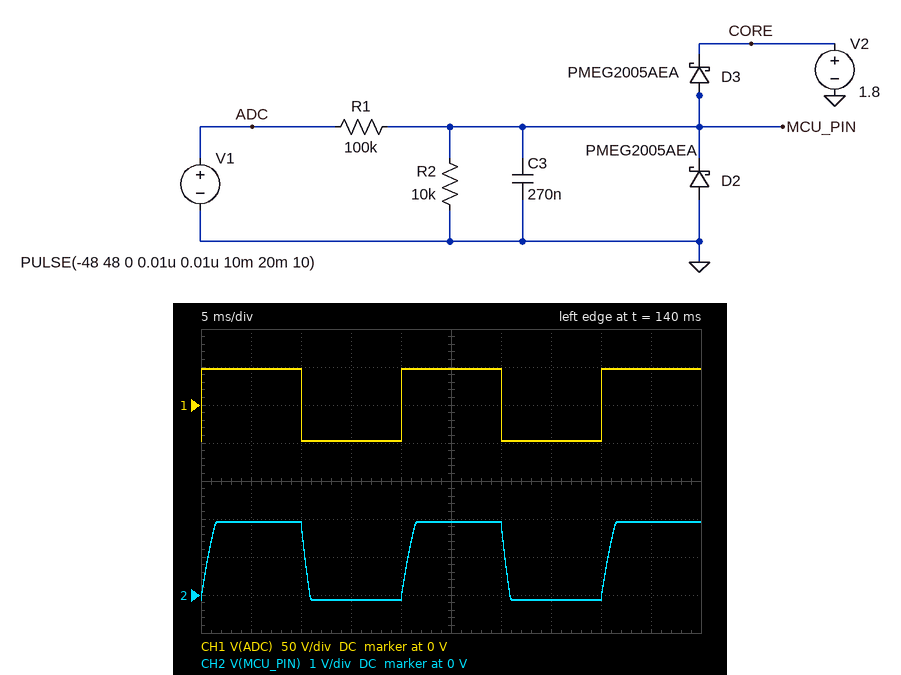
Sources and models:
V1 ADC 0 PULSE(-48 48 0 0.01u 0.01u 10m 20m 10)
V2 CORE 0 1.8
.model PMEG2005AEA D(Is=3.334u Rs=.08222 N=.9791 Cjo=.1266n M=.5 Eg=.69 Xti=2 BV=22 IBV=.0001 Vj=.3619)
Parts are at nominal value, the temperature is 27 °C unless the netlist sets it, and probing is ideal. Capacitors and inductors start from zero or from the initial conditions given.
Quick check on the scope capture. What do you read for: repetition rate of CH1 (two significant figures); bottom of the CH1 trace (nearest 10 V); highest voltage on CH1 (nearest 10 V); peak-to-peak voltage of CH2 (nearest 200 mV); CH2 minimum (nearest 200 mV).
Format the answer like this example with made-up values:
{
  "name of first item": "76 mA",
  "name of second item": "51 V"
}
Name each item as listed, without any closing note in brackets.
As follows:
{
  "repetition rate of CH1": "50 Hz",
  "bottom of the CH1 trace": "-50 V",
  "highest voltage on CH1": "50 V",
  "peak-to-peak voltage of CH2": "2.0 V",
  "CH2 minimum": "-200 mV"
}
